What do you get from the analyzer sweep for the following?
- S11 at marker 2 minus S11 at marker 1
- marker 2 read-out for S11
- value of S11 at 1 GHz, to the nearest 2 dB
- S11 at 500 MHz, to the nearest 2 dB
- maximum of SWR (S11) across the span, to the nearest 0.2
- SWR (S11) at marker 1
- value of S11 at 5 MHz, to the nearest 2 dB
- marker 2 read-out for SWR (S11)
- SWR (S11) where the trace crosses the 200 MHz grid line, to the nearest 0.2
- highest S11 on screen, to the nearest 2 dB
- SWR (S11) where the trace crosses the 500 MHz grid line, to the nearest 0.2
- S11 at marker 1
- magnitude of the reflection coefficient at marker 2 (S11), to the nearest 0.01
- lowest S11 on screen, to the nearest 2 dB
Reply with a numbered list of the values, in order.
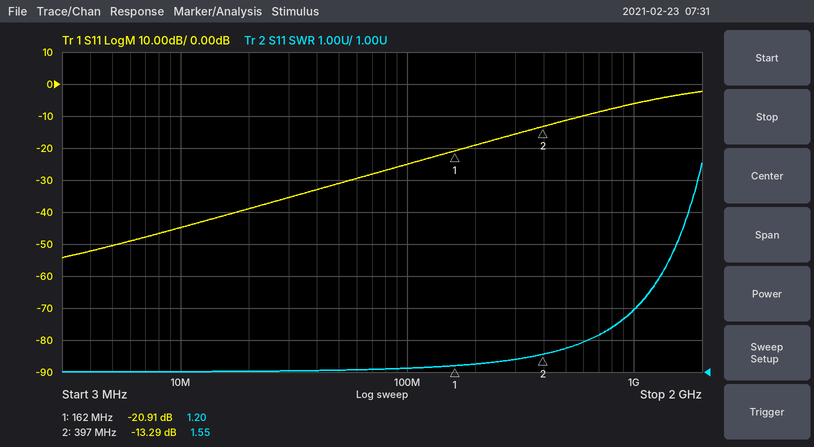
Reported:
1. 7.62 dB
2. -13.29 dB
3. -6 dB
4. -12 dB
5. 7.6
6. 1.20
7. -50 dB
8. 1.55
9. 1.2
10. -2 dB
11. 1.8
12. -20.91 dB
13. 0.22
14. -54 dB
